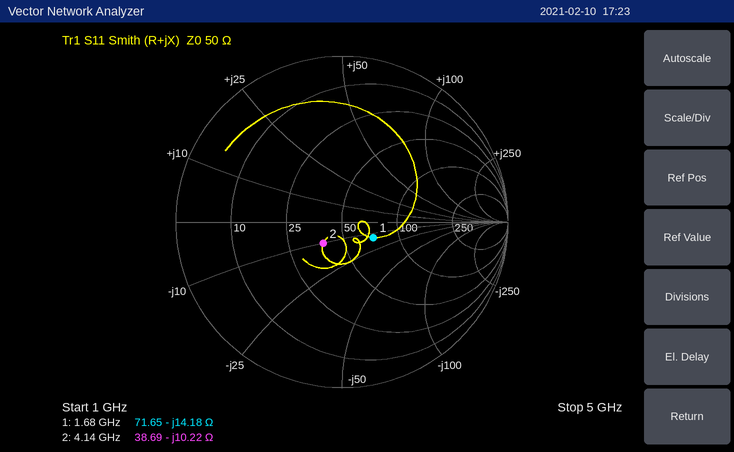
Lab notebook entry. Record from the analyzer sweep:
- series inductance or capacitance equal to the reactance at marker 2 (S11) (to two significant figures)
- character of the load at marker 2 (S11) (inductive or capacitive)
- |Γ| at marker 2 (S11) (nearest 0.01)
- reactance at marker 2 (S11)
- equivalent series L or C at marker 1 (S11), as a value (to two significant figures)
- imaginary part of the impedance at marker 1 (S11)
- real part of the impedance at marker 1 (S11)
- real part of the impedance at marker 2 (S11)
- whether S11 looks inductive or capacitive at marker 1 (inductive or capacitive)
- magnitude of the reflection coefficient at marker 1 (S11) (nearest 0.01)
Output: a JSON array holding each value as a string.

["3.8 pF", "capacitive", "0.17", "-10.22 Ω", "6.7 pF", "-14.18 Ω", "71.65 Ω", "38.69 Ω", "capacitive", "0.21"]
